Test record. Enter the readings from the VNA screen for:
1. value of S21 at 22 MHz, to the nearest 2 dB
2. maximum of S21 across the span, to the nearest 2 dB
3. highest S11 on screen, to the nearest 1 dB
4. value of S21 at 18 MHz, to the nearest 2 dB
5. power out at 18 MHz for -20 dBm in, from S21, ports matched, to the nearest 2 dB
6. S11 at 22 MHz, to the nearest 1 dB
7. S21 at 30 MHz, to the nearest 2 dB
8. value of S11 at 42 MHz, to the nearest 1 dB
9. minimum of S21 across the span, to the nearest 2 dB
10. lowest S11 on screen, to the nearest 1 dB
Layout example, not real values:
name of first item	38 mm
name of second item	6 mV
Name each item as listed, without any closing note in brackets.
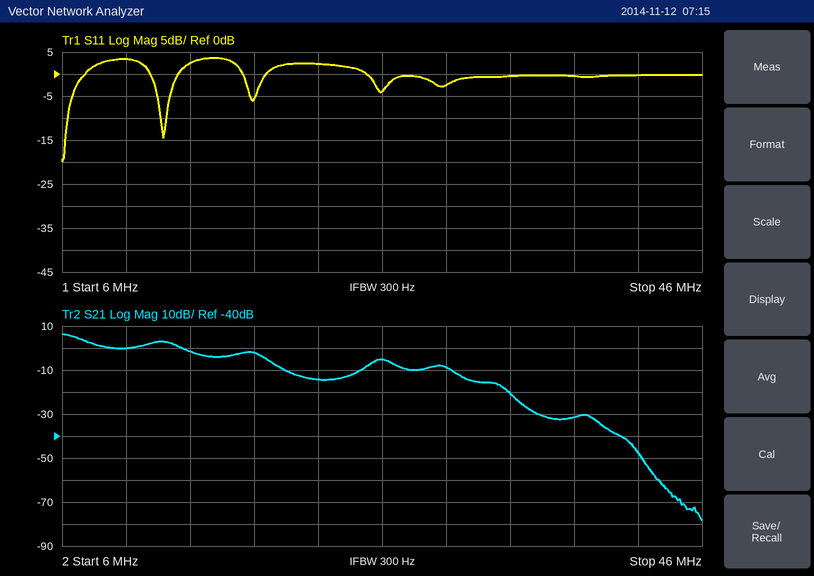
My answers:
value of S21 at 22 MHz, to the nearest 2 dB	-14 dB
maximum of S21 across the span, to the nearest 2 dB	6 dB
highest S11 on screen, to the nearest 1 dB	4 dB
value of S21 at 18 MHz, to the nearest 2 dB	-2 dB
power out at 18 MHz for -20 dBm in, from S21, ports matched, to the nearest 2 dB	-22 dBm
S11 at 22 MHz, to the nearest 1 dB	2 dB
S21 at 30 MHz, to the nearest 2 dB	-8 dB
value of S11 at 42 MHz, to the nearest 1 dB	0 dB
minimum of S21 across the span, to the nearest 2 dB	-78 dB
lowest S11 on screen, to the nearest 1 dB	-20 dB
